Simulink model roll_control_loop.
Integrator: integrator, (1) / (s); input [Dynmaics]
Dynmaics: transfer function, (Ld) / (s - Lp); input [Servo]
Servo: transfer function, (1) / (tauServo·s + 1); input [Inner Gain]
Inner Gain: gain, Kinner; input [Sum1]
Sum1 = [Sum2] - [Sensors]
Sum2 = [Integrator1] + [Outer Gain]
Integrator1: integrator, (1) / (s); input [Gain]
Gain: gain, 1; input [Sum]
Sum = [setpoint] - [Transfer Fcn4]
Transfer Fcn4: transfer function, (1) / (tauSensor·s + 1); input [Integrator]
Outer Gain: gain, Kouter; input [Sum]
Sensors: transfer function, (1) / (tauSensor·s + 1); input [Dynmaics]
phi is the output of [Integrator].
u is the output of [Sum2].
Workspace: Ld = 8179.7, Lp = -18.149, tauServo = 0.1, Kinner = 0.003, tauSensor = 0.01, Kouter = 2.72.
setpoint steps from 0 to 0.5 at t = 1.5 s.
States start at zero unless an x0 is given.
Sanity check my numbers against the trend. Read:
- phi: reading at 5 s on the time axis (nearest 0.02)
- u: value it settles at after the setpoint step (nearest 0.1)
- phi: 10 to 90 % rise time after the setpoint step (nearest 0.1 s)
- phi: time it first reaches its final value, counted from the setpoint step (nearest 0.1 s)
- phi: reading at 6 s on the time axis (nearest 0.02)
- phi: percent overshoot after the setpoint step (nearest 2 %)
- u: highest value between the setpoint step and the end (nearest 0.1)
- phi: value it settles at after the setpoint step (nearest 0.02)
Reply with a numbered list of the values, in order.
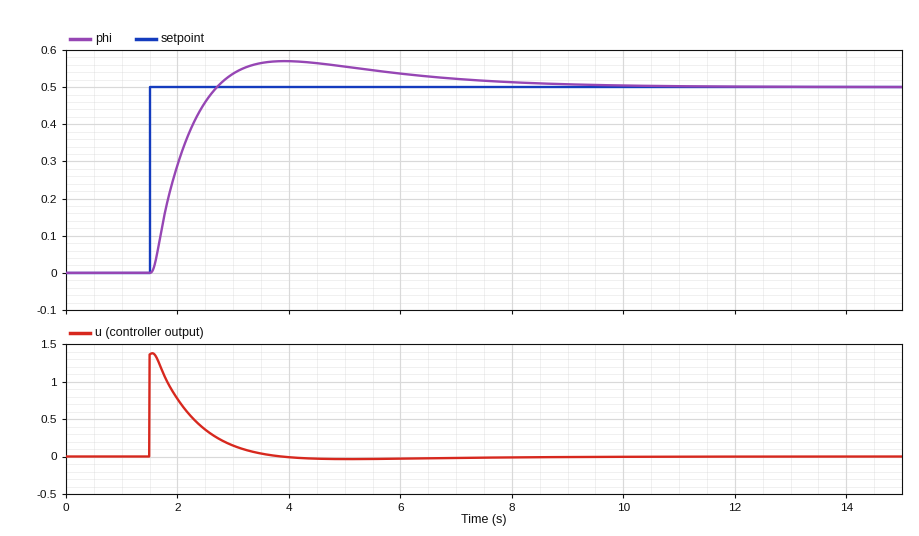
1. 0.56
2. 0.0
3. 0.8 s
4. 1.2 s
5. 0.54
6. 14 %
7. 1.4
8. 0.50
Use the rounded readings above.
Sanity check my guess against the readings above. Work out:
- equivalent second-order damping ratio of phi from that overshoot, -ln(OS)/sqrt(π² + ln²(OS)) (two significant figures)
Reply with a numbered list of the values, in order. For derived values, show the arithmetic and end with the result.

1. ln(0.14) = -1.966; 1.966 / sqrt(9.870 + 3.866) = 0.53
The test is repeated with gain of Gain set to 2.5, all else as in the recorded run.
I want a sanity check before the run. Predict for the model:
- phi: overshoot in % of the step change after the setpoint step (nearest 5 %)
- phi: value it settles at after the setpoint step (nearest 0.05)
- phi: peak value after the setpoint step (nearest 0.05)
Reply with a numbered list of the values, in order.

1. 25 %
2. 0.50
3. 0.65
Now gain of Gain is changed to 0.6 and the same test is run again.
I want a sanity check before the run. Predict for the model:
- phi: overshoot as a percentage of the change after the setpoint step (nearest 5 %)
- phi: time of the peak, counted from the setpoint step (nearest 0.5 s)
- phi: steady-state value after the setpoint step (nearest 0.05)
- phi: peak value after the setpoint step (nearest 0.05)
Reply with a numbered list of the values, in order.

1. 10 %
2. 3.0 s
3. 0.50
4. 0.55
